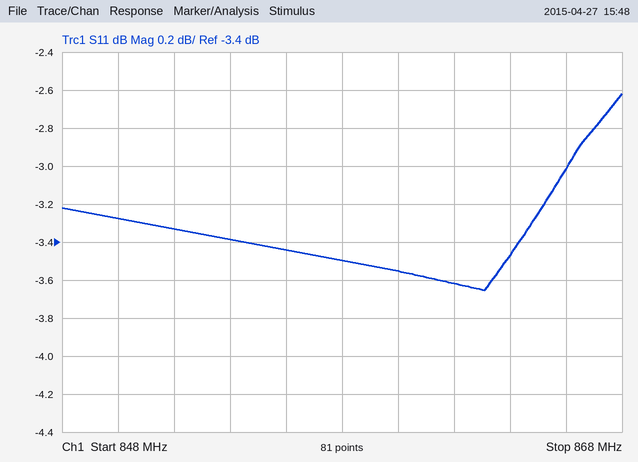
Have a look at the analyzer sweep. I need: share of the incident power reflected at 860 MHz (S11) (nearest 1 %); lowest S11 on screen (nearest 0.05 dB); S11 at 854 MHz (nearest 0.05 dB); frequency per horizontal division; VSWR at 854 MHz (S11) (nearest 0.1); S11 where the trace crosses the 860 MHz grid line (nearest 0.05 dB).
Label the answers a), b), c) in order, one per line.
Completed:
a) 44 %
b) -3.65 dB
c) -3.40 dB
d) 2 MHz
e) 5.2
f) -3.55 dB
